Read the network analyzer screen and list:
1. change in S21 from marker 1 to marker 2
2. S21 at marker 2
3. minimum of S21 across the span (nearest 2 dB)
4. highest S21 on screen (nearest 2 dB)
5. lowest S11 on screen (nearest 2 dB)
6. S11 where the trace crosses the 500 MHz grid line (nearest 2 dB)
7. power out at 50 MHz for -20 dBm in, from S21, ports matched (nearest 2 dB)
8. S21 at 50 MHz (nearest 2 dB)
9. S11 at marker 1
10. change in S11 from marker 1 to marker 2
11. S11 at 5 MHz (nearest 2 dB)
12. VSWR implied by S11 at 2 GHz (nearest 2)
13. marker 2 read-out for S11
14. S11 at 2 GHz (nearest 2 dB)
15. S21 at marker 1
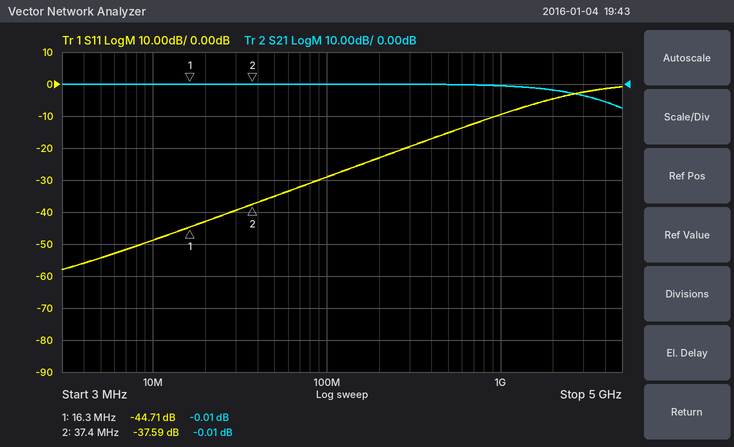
0.00 dB
-0.01 dB
-8 dB
0 dB
-58 dB
-16 dB
-20 dBm
0 dB
-44.71 dB
7.12 dB
-54 dB
4
-37.59 dB
-4 dB
-0.01 dB
